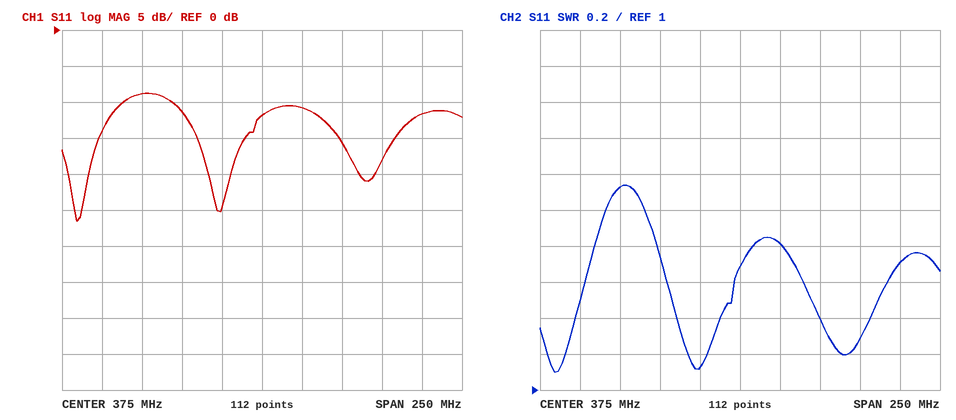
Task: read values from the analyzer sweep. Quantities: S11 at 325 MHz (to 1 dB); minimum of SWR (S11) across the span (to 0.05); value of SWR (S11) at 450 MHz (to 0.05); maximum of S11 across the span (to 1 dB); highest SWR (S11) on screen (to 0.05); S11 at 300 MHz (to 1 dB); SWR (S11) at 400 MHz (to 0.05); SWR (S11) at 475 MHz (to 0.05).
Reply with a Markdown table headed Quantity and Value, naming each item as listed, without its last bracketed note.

| Quantity | Value |
|---|---|
| S11 at 325 MHz | -11 dB |
| minimum of SWR (S11) across the span | 1.10 |
| value of SWR (S11) at 450 MHz | 1.30 |
| maximum of S11 across the span | -9 dB |
| highest SWR (S11) on screen | 2.15 |
| S11 at 300 MHz | -9 dB |
| SWR (S11) at 400 MHz | 1.80 |
| SWR (S11) at 475 MHz | 1.70 |
